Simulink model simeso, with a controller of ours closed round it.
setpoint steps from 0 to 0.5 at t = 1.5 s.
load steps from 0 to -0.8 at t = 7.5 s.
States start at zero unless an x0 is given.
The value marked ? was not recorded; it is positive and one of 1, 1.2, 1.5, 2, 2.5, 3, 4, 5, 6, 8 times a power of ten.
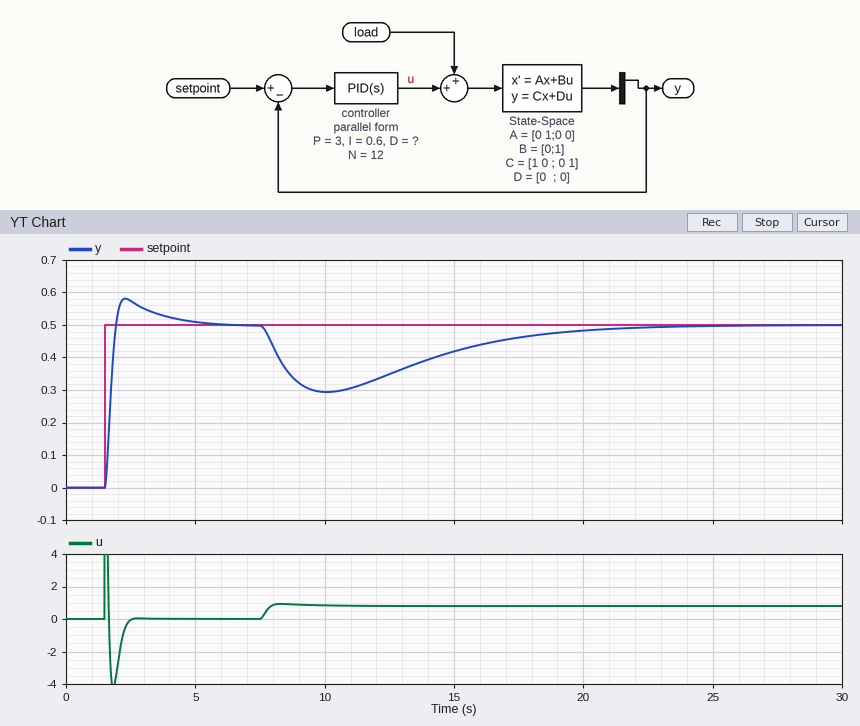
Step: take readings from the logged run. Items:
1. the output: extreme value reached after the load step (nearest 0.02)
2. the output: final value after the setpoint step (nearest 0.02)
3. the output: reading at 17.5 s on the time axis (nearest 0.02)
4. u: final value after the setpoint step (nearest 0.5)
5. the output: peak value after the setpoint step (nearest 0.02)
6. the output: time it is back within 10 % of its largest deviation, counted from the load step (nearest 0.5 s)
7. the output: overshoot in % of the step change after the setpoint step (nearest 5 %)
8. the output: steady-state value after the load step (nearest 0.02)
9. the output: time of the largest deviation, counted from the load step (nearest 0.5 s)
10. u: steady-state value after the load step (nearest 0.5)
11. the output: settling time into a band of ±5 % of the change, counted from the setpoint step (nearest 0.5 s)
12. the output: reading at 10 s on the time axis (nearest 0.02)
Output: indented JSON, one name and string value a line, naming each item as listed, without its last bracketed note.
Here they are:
{
  "the output: extreme value reached after the load step": "0.30",
  "the output: final value after the setpoint step": "0.50",
  "the output: reading at 17.5 s on the time axis": "0.46",
  "u: final value after the setpoint step": "0.0",
  "the output: peak value after the setpoint step": "0.58",
  "the output: time it is back within 10 % of its largest deviation, counted from the load step": "12.0 s",
  "the output: overshoot in % of the step change after the setpoint step": "15 %",
  "the output: steady-state value after the load step": "0.50",
  "the output: time of the largest deviation, counted from the load step": "2.5 s",
  "u: steady-state value after the load step": "1.0",
  "the output: settling time into a band of ±5 % of the change, counted from the setpoint step": "2.5 s",
  "the output: reading at 10 s on the time axis": "0.30"
}
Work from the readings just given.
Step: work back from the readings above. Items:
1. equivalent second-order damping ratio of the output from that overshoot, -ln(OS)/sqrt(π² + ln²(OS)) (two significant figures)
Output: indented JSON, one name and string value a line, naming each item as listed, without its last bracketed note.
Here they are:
{
  "equivalent second-order damping ratio of the output from that overshoot, -ln(OS)/sqrt(π² + ln²(OS))": "0.52"
}
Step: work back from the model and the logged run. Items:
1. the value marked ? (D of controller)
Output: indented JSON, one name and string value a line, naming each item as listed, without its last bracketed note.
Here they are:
{
  "the value marked ?": "4"
}
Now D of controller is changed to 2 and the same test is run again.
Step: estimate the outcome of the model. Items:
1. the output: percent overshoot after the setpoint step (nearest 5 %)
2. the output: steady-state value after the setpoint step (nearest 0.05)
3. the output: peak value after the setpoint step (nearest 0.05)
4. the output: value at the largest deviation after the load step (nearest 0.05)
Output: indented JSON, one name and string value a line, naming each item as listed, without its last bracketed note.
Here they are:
{
  "the output: percent overshoot after the setpoint step": "35 %",
  "the output: steady-state value after the setpoint step": "0.50",
  "the output: peak value after the setpoint step": "0.65",
  "the output: value at the largest deviation after the load step": "0.25"
}
